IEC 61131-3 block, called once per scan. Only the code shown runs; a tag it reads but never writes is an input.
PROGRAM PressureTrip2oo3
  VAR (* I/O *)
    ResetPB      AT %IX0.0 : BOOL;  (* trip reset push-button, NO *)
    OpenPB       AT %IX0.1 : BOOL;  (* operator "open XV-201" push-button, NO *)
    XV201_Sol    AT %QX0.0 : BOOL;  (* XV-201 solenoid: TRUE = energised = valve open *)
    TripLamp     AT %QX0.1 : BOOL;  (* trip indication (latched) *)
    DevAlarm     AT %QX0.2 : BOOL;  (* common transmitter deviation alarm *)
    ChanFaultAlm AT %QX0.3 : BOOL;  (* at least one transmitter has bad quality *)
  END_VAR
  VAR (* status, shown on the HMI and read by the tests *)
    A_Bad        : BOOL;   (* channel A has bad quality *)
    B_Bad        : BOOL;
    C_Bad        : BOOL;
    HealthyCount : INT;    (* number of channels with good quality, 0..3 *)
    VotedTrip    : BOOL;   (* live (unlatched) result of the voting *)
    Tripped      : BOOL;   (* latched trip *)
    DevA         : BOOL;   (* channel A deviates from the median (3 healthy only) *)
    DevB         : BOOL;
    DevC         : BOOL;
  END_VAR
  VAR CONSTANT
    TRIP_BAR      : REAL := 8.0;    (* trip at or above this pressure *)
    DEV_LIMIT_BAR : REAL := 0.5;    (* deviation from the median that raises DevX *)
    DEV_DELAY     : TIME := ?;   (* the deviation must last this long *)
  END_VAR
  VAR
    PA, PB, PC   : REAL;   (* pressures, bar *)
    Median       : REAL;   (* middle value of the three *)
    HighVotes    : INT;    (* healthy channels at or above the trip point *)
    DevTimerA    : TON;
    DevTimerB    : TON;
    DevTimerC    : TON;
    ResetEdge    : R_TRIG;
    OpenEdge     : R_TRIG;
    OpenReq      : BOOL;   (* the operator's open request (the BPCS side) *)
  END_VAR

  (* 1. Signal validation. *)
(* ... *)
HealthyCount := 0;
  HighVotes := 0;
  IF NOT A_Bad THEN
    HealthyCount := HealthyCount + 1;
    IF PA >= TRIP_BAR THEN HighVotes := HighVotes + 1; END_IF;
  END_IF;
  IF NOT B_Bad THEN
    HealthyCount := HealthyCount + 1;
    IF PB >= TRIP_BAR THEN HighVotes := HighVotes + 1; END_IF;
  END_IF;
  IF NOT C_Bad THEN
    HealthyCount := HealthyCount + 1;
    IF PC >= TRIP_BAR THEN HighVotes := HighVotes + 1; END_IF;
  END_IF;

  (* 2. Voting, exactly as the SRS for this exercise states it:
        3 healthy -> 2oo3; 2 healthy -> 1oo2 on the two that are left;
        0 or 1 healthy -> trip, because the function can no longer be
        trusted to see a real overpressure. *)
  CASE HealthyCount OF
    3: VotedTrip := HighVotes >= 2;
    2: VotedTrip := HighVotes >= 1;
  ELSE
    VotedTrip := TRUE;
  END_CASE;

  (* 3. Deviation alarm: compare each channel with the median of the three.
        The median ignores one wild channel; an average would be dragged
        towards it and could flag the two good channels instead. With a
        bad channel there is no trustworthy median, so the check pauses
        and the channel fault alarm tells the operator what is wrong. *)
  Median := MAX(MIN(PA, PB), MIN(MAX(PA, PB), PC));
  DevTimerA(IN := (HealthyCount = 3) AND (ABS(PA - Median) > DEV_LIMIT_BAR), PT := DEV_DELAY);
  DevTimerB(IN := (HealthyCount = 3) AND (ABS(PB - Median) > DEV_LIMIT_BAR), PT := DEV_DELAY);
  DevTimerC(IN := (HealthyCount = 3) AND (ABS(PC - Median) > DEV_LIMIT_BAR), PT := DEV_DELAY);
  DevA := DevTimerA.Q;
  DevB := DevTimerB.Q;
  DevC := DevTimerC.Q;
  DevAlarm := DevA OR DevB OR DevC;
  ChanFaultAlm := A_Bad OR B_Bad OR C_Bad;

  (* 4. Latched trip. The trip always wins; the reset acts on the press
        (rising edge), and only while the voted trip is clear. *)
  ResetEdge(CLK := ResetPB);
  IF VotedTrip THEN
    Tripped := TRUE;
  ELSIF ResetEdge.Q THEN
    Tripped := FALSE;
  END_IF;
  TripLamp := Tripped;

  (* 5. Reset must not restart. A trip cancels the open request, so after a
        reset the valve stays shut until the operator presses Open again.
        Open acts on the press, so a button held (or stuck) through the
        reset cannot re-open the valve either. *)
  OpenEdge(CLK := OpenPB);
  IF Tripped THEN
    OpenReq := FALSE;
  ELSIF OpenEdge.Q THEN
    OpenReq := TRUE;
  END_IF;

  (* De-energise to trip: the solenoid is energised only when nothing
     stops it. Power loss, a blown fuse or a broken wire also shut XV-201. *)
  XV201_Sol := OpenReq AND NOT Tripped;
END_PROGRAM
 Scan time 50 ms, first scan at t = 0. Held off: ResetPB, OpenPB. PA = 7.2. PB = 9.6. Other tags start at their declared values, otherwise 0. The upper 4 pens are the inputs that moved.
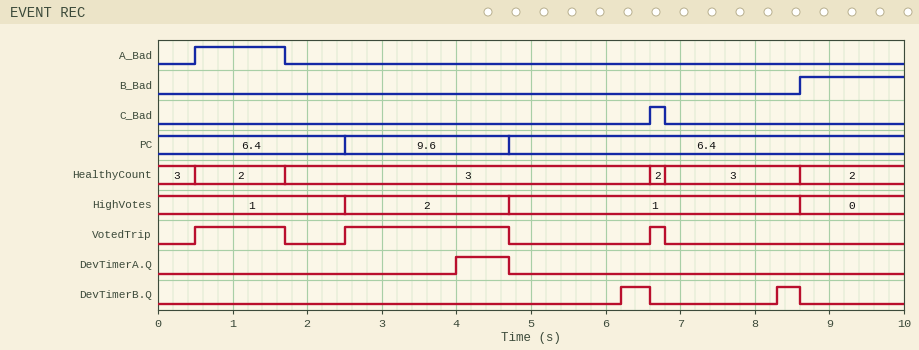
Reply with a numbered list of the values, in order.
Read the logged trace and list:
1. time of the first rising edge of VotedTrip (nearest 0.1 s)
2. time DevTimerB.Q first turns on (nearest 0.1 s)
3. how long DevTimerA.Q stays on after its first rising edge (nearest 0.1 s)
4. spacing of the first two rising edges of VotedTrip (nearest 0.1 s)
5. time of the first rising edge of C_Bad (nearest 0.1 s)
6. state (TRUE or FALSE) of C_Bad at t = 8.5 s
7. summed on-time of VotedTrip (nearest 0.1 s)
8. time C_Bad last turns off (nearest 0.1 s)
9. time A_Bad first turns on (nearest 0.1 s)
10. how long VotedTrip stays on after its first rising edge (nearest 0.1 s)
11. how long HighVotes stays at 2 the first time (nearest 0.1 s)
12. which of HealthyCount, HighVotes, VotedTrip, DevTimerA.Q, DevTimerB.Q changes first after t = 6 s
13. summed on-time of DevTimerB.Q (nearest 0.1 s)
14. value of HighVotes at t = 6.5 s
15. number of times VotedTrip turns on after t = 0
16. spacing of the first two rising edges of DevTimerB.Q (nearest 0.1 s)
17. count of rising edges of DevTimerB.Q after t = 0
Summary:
1. 0.5 s
2. 6.2 s
3. 0.7 s
4. 2.0 s
5. 6.6 s
6. FALSE
7. 3.6 s
8. 6.8 s
9. 0.5 s
10. 1.2 s
11. 2.2 s
12. DevTimerB.Q
13. 0.7 s
14. 1
15. 3
16. 2.1 s
17. 2
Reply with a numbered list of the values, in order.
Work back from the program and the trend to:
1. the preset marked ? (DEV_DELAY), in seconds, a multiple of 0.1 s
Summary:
1. 1.5 s
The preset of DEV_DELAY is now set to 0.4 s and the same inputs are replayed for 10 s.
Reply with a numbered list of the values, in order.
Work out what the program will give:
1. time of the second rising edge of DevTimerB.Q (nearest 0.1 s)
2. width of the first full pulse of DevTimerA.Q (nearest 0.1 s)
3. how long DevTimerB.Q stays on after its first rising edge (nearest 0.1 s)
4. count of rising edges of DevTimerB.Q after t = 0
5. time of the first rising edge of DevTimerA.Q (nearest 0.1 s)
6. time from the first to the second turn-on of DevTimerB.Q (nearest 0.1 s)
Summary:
1. 2.1 s
2. 1.8 s
3. 0.1 s
4. 4
5. 2.9 s
6. 1.7 s
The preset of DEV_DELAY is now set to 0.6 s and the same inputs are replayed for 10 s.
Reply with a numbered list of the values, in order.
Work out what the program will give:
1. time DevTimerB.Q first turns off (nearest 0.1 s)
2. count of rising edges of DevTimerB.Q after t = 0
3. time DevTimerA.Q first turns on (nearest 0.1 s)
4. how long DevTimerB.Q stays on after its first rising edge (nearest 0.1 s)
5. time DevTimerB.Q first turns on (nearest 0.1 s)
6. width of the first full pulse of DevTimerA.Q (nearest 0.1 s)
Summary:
1. 2.5 s
2. 3
3. 3.1 s
4. 0.2 s
5. 2.3 s
6. 1.6 s
